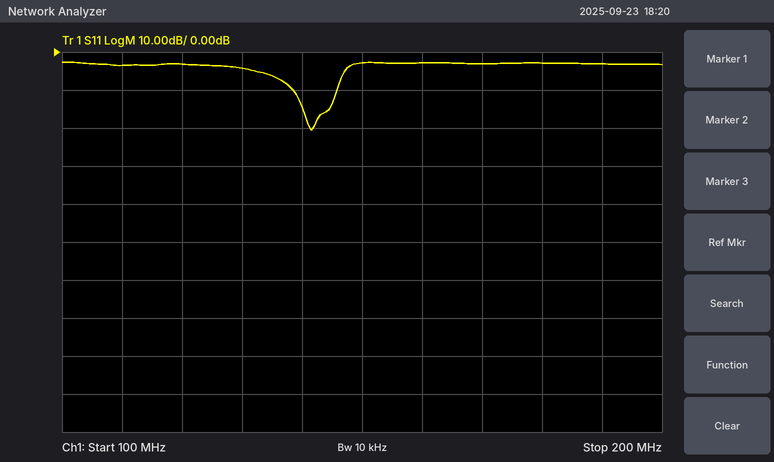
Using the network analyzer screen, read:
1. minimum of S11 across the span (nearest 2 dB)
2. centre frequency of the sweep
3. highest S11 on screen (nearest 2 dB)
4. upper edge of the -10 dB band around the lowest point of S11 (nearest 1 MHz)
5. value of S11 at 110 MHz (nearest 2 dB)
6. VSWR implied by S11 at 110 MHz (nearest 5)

-20 dB
150 MHz
-2 dB
146 MHz
-4 dB
5
